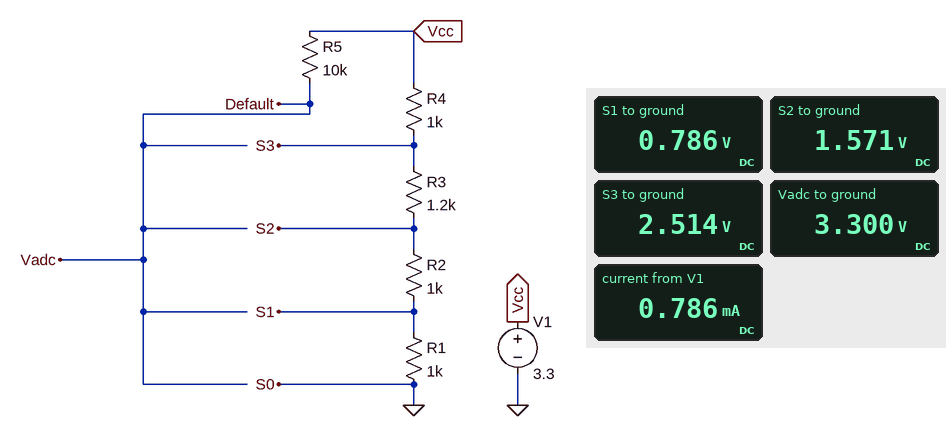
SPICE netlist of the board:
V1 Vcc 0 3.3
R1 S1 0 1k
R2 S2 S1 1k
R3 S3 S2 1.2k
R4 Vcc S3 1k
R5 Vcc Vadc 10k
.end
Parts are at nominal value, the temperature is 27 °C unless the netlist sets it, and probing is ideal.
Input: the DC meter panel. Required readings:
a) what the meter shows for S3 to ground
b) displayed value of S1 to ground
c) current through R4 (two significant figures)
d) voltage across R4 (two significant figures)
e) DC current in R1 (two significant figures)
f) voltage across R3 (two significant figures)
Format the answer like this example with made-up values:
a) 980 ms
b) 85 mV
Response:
a) 2.514 V
b) 0.786 V
c) 790 µA
d) 790 mV
e) 790 µA
f) 940 mV
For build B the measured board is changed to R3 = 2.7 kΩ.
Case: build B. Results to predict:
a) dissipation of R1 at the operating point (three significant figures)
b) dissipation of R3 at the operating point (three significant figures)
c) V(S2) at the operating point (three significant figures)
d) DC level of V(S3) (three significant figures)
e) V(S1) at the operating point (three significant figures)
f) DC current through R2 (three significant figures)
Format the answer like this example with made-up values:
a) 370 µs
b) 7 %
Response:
a) 335 µW
b) 905 µW
c) 1.16 V
d) 2.72 V
e) 579 mV
f) 579 µA
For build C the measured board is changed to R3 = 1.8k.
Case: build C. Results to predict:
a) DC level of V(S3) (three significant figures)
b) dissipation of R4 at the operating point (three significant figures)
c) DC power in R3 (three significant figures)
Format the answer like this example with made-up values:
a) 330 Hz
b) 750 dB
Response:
a) 2.61 V
b) 473 µW
c) 851 µW
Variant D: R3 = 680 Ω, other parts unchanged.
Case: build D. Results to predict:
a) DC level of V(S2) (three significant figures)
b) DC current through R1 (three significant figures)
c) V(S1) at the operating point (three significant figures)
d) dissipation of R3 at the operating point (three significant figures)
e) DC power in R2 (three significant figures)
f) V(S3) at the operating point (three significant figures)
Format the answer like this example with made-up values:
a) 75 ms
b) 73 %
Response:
a) 1.79 V
b) 897 µA
c) 897 mV
d) 547 µW
e) 804 µW
f) 2.40 V
